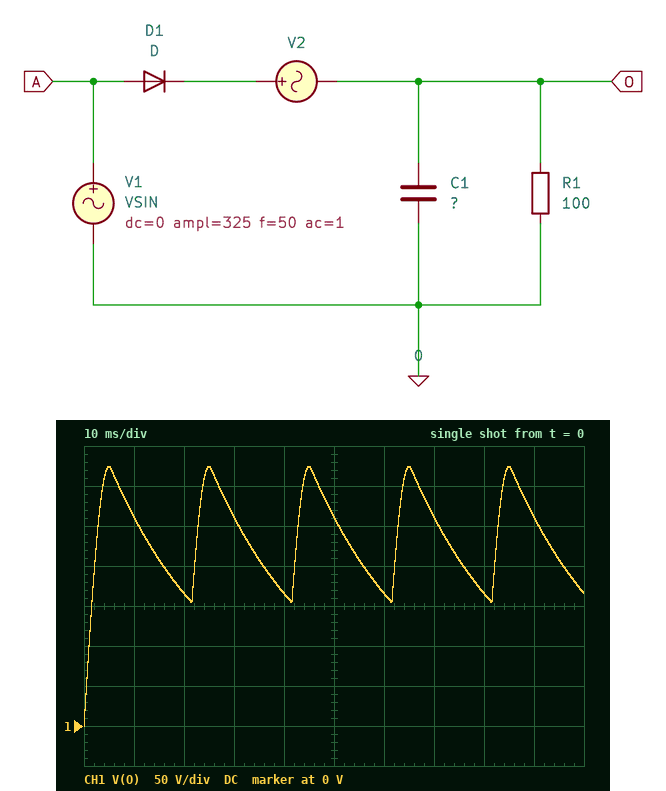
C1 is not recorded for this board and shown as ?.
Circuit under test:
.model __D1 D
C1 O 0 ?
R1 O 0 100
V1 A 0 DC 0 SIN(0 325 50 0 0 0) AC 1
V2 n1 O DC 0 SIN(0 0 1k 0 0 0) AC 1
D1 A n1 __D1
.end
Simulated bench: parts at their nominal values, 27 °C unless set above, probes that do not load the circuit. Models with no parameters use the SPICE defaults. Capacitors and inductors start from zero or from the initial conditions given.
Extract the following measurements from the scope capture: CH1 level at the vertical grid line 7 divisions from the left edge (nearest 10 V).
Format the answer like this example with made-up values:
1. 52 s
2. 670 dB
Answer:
1. 260 V
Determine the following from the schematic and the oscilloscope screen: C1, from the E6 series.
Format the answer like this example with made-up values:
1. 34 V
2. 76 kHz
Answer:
1. 220 µF
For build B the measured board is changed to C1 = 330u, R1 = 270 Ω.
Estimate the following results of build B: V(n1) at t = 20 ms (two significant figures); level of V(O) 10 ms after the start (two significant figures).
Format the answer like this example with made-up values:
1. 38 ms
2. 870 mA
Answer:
1. 270 V
2. 310 V
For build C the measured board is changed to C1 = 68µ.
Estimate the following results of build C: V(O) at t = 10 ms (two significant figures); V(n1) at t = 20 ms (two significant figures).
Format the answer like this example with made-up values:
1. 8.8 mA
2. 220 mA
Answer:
1. 170 V
2. 40 V
